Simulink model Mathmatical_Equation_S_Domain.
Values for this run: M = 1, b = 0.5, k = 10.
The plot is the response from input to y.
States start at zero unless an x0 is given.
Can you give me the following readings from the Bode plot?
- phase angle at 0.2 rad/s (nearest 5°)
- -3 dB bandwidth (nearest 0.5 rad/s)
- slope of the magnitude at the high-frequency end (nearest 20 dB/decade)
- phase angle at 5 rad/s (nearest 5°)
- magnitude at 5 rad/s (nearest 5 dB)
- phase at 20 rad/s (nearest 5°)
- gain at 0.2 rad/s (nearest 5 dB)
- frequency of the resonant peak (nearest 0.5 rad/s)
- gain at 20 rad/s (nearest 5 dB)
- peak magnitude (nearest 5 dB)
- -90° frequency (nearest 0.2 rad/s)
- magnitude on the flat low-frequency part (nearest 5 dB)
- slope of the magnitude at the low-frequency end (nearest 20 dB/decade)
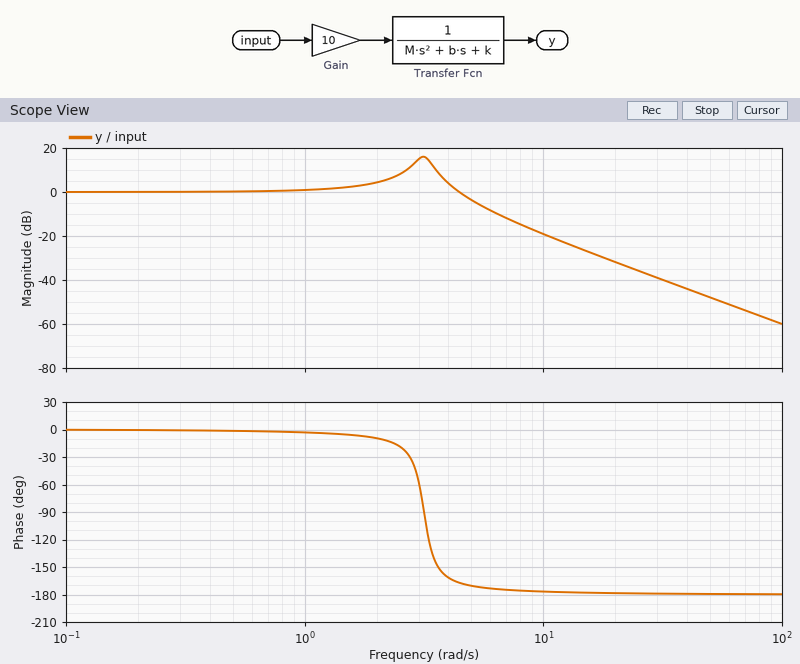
0°
5.0 rad/s
-40 dB/decade
-170°
-5 dB
-180°
0 dB
3.0 rad/s
-30 dB
15 dB
3.2 rad/s
0 dB
0 dB/decade
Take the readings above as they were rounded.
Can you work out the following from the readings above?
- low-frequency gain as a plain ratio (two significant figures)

1.0
